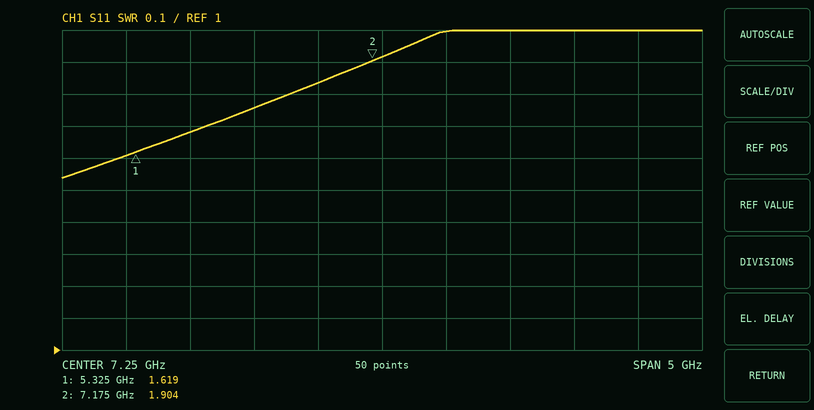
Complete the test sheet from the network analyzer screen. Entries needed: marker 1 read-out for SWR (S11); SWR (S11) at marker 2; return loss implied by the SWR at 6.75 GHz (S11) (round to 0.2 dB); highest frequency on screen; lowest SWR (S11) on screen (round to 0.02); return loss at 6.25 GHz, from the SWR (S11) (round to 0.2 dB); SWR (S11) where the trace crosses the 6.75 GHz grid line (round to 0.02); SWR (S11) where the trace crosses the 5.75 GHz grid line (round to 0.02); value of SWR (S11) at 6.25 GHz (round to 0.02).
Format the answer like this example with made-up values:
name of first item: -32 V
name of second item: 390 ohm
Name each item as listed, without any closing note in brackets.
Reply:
marker 1 read-out for SWR: 1.619
SWR (S11) at marker 2: 1.904
return loss implied by the SWR at 6.75 GHz (S11): 10.6 dB
highest frequency on screen: 9.75 GHz
lowest SWR (S11) on screen: 1.54
return loss at 6.25 GHz, from the SWR (S11): 11.2 dB
SWR (S11) where the trace crosses the 6.75 GHz grid line: 1.84
SWR (S11) where the trace crosses the 5.75 GHz grid line: 1.68
value of SWR (S11) at 6.25 GHz: 1.76
